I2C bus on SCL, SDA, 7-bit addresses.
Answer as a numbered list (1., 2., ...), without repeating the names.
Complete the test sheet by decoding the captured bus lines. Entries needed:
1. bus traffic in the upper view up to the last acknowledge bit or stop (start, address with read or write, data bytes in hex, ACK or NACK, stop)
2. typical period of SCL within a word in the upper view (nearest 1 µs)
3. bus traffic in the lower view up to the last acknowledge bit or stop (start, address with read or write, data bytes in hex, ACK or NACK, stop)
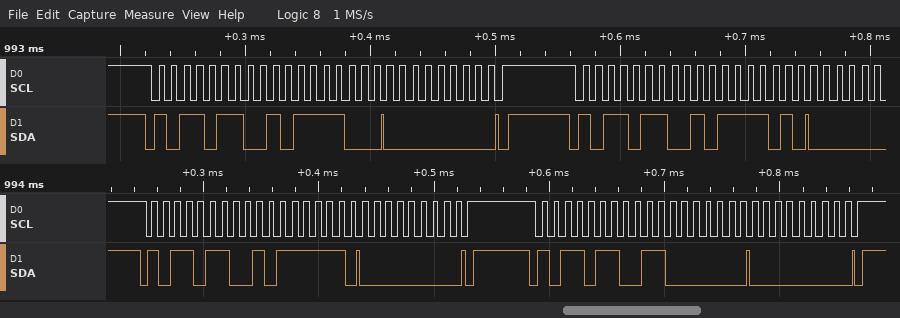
1. start, address 5B write ACK, BC ACK, 00 ACK, stop, start, address 5B write ACK, BD ACK
2. 10 µs
3. start, address 5B write ACK, BF ACK, 00 ACK, stop, start, address 5B write ACK, C0 ACK, 00 ACK, stop
